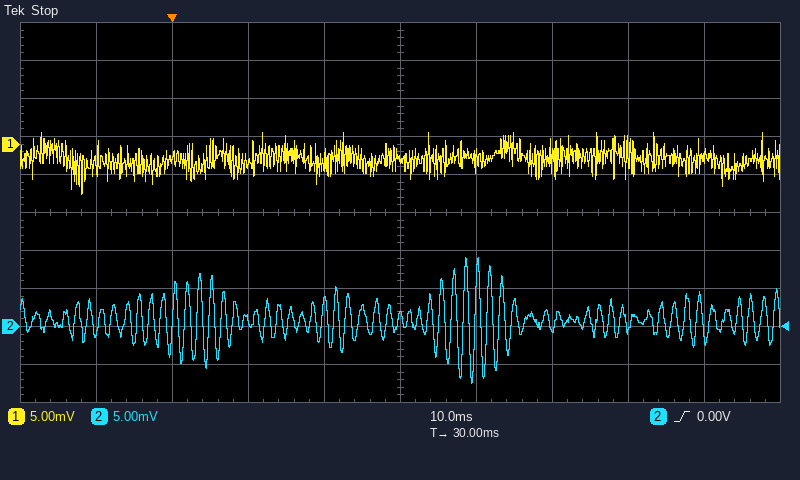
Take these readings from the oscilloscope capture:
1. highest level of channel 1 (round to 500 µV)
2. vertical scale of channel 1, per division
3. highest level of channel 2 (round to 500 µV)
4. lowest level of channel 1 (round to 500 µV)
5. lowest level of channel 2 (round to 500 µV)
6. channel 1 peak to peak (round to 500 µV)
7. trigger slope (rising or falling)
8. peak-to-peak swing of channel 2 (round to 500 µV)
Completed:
1.5 mV
5 mV
9.0 mV
-6.5 mV
-7.5 mV
8.0 mV
rising
16.5 mV
